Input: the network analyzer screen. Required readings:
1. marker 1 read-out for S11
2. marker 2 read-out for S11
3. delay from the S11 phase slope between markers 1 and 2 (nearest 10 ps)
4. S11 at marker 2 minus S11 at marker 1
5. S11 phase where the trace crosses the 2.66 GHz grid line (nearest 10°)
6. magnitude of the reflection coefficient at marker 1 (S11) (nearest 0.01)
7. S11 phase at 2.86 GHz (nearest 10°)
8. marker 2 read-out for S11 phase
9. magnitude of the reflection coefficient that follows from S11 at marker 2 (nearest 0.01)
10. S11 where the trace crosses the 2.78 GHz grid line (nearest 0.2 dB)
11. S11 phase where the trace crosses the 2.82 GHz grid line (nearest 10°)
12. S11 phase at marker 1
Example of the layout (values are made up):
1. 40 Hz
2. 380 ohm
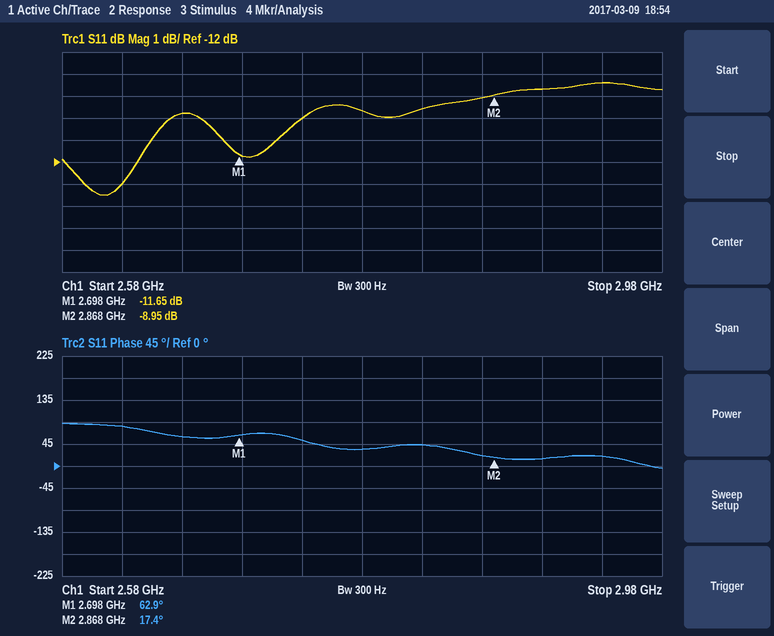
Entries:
1. -11.65 dB
2. -8.95 dB
3. 740 ps
4. 2.70 dB
5. 60°
6. 0.26
7. 20°
8. 17.4°
9. 0.36
10. -9.6 dB
11. 40°
12. 62.9°
